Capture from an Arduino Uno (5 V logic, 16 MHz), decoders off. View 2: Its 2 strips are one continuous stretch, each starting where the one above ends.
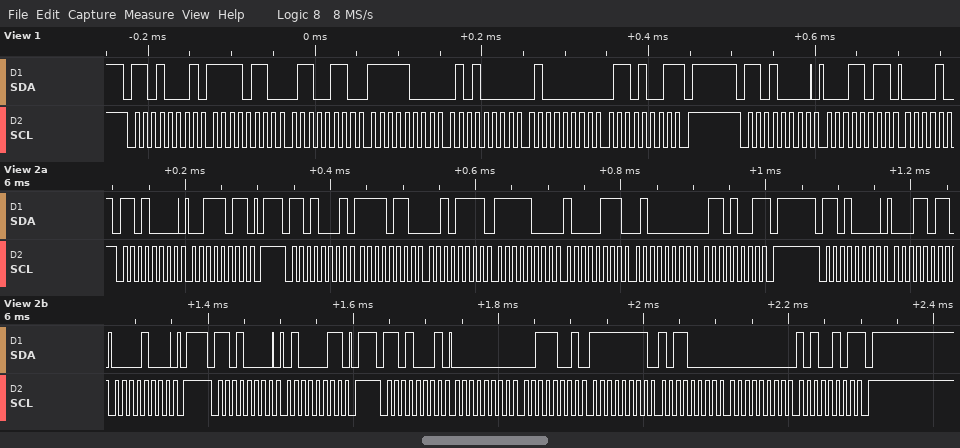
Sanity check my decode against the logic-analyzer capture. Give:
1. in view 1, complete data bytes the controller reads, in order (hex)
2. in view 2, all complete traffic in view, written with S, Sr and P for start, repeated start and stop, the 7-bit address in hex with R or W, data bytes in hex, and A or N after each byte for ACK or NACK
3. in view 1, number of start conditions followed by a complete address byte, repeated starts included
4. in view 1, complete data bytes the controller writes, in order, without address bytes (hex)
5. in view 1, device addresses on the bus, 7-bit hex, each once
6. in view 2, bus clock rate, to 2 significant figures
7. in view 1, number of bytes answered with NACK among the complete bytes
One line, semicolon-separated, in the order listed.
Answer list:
F6 66 F8 50 40 69; S 68W A 3B A P S 68R A F6 A 2F A F8 A 87 A 40 A 69 N P S 68W A 1B A 08 A P S 68W A 43 A P S 68R A 00 A 39 A FF A B0 A 00 A A5 N P; 2; 1B; 0x68; 100 kHz; 1
